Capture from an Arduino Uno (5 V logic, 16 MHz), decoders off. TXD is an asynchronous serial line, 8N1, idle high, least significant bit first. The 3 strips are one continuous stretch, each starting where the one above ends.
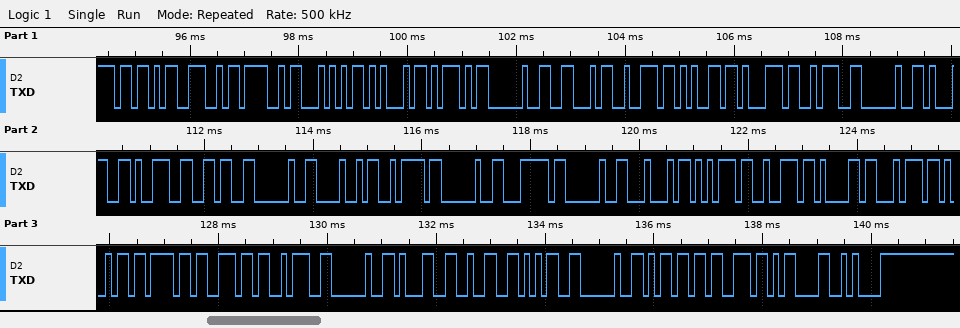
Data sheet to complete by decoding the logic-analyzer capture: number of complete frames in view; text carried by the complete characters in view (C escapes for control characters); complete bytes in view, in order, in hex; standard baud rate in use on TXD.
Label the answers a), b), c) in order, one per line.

a) 40
b) "[NOTE] Freq: 196 Hz | Duration: 125 ms\r\n"
c) 5B 4E 4F 54 45 5D 20 46 72 65 71 3A 20 31 39 36 20 48 7A 20 7C 20 44 75 72 61 74 69 6F 6E 3A 20 31 32 35 20 6D 73 0D 0A
d) 9600 baud
